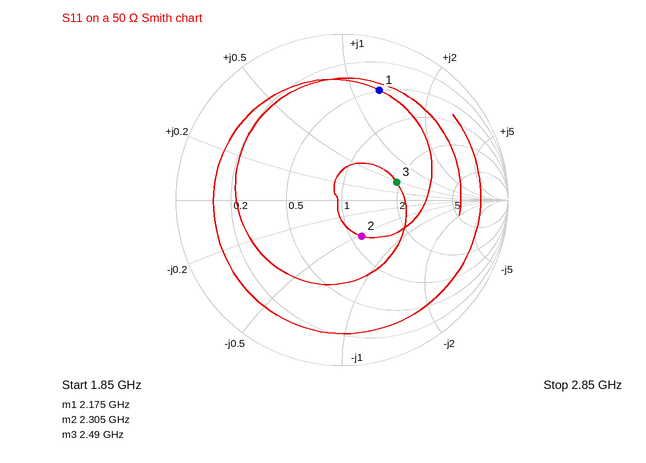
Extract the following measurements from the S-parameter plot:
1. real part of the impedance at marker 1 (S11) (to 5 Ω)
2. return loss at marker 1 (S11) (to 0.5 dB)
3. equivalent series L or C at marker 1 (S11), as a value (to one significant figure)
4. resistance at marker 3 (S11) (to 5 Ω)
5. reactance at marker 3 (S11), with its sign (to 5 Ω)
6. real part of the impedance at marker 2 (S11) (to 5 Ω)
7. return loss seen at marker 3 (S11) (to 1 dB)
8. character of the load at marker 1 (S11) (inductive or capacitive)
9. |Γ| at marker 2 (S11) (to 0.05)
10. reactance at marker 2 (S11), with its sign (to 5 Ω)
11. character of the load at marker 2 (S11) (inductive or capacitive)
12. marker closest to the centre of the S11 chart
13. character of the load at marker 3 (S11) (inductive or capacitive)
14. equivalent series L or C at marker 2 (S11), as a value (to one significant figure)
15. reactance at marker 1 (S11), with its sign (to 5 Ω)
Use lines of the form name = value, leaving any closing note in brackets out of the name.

real part of the impedance at marker 1 (S11) = 25 Ω
return loss at marker 1 (S11) = 3.0 dB
equivalent series L or C at marker 1 (S11), as a value = 5 nH
resistance at marker 3 (S11) = 95 Ω
reactance at marker 3 (S11), with its sign = +25 Ω
real part of the impedance at marker 2 (S11) = 55 Ω
return loss seen at marker 3 (S11) = 9 dB
character of the load at marker 1 (S11) = inductive
|Γ| at marker 2 (S11) = 0.25
reactance at marker 2 (S11), with its sign = -25 Ω
character of the load at marker 2 (S11) = capacitive
marker closest to the centre of the S11 chart = marker 2
character of the load at marker 3 (S11) = inductive
equivalent series L or C at marker 2 (S11), as a value = 3 pF
reactance at marker 1 (S11), with its sign = +65 Ω
